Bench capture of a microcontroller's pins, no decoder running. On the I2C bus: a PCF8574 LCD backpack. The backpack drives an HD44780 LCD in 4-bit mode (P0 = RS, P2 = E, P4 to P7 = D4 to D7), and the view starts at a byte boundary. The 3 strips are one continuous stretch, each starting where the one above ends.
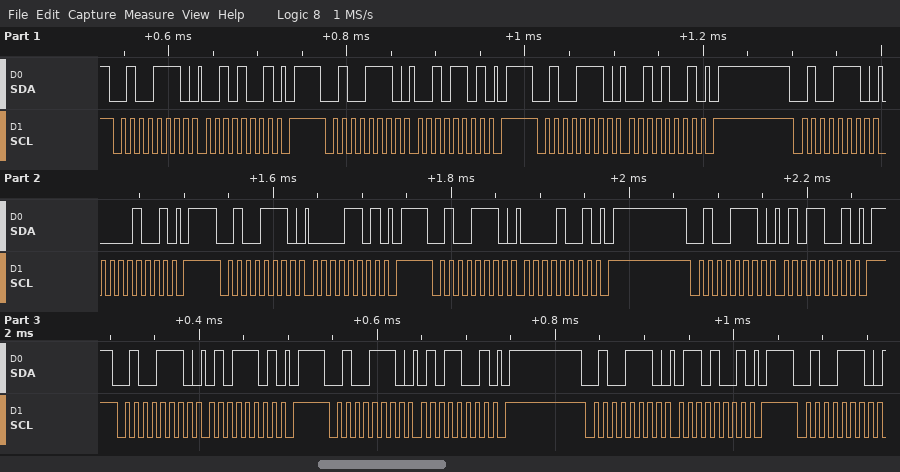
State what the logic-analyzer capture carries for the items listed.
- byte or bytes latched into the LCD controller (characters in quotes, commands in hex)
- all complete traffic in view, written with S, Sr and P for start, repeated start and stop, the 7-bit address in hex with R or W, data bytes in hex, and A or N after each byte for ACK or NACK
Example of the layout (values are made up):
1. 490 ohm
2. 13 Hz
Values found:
1. ' '
2. S 27W A 29 A P S 27W A 2D A P S 27W A 29 A P S 27W A 09 A P S 27W A 0D A P S 27W A 09 A P S 27W A 59 A P S 27W A 5D A P S 27W A 59 A P S 27W A 69 A P S 27W A
